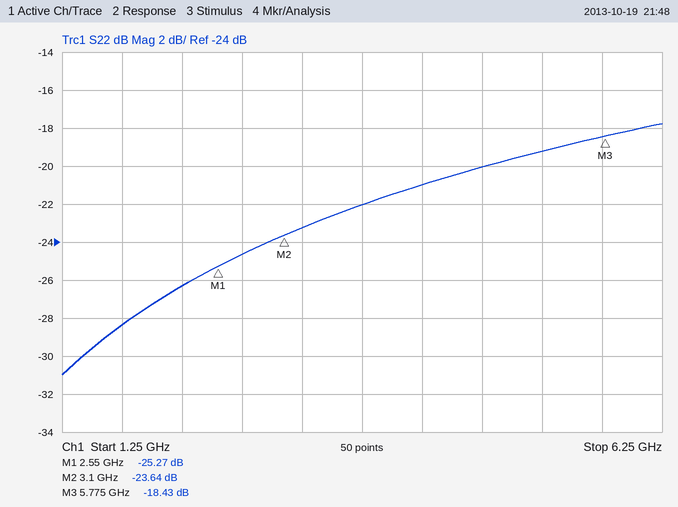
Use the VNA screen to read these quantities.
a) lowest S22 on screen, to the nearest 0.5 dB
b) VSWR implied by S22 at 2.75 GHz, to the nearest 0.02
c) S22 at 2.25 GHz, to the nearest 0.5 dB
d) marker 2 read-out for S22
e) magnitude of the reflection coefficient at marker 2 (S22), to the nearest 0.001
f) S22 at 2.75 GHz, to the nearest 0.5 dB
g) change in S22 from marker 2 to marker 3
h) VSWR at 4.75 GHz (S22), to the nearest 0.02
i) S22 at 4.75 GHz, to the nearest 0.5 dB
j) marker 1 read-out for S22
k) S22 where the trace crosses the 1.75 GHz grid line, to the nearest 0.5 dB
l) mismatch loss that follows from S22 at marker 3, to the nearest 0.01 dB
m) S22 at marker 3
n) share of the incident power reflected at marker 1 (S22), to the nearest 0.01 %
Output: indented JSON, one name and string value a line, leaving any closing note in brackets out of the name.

{
  "lowest S22 on screen, to the nearest 0.5 dB": "-31.0 dB",
  "VSWR implied by S22 at 2.75 GHz, to the nearest 0.02": "1.12",
  "S22 at 2.25 GHz, to the nearest 0.5 dB": "-26.5 dB",
  "marker 2 read-out for S22": "-23.64 dB",
  "magnitude of the reflection coefficient at marker 2 (S22), to the nearest 0.001": "0.066",
  "S22 at 2.75 GHz, to the nearest 0.5 dB": "-24.5 dB",
  "change in S22 from marker 2 to marker 3": "5.21 dB",
  "VSWR at 4.75 GHz (S22), to the nearest 0.02": "1.22",
  "S22 at 4.75 GHz, to the nearest 0.5 dB": "-20.0 dB",
  "marker 1 read-out for S22": "-25.27 dB",
  "S22 where the trace crosses the 1.75 GHz grid line, to the nearest 0.5 dB": "-28.5 dB",
  "mismatch loss that follows from S22 at marker 3, to the nearest 0.01 dB": "0.06 dB",
  "S22 at marker 3": "-18.43 dB",
  "share of the incident power reflected at marker 1 (S22), to the nearest 0.01 %": "0.30 %"
}
